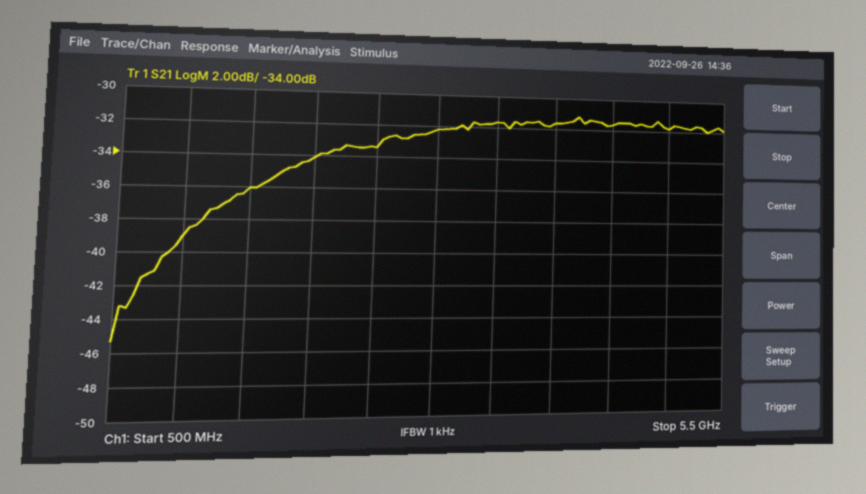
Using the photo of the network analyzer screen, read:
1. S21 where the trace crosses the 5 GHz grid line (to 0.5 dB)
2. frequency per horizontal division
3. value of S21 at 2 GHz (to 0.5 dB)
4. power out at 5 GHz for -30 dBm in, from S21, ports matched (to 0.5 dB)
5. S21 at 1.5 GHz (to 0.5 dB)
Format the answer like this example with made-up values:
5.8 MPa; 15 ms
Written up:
-32.0 dB; 500 MHz; -34.0 dB; -62.0 dBm; -36.0 dB
